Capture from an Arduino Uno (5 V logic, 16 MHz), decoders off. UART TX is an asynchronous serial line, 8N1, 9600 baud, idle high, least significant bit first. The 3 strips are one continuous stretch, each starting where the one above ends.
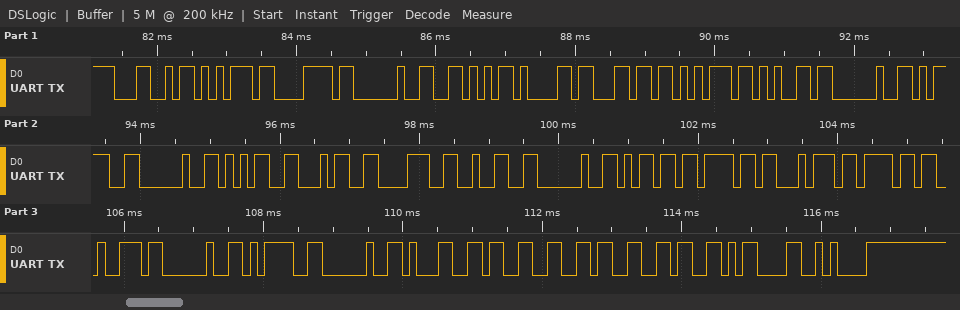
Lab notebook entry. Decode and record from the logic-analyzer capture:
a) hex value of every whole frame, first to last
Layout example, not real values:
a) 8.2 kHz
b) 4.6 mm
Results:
a) 4C 75 78 20 56 61 6C 75 65 20 3D 20 35 34 38 32 20 6D 6F 74 6F 72 20 3D 20 31 33 36 36 0D 0A
